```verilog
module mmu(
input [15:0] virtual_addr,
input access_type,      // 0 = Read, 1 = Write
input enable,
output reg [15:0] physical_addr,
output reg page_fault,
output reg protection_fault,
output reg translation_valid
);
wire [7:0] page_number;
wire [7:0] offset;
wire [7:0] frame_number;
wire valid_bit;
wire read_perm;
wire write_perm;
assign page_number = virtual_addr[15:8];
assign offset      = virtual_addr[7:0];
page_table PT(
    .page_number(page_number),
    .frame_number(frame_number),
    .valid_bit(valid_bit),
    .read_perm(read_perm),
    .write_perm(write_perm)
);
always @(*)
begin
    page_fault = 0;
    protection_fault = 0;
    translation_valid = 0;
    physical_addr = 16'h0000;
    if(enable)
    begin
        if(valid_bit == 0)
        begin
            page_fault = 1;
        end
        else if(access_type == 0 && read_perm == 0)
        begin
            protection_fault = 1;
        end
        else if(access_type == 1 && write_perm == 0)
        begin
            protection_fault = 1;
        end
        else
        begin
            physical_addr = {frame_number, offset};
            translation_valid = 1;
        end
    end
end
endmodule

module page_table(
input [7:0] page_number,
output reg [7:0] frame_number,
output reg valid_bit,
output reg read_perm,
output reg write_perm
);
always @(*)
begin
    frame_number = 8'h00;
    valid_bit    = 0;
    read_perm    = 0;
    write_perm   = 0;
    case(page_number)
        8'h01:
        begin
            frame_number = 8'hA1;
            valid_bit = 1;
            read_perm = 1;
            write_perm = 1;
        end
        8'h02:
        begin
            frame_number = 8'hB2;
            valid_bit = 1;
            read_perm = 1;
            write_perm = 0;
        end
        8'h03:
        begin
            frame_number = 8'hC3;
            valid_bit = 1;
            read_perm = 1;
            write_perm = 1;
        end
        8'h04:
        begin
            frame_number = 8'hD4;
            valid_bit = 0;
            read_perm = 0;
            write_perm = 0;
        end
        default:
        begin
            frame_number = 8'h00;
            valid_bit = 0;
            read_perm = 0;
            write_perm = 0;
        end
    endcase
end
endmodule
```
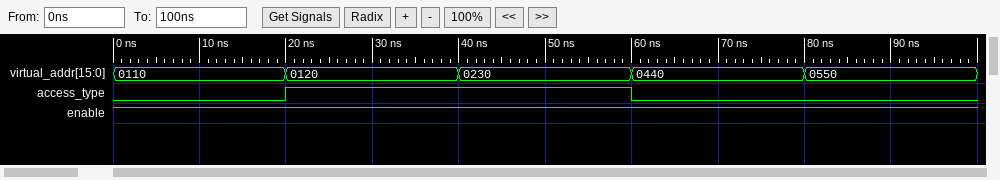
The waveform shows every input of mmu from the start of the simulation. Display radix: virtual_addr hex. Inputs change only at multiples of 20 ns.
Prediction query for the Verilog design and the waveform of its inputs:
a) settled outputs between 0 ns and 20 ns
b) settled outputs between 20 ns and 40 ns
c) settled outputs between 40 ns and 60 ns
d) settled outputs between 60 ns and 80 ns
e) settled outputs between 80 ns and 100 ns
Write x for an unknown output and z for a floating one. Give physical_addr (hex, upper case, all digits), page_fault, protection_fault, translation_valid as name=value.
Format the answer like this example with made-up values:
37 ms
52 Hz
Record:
physical_addr=A110, page_fault=0, protection_fault=0, translation_valid=1
physical_addr=A120, page_fault=0, protection_fault=0, translation_valid=1
physical_addr=0000, page_fault=0, protection_fault=1, translation_valid=0
physical_addr=0000, page_fault=1, protection_fault=0, translation_valid=0
physical_addr=0000, page_fault=1, protection_fault=0, translation_valid=0
